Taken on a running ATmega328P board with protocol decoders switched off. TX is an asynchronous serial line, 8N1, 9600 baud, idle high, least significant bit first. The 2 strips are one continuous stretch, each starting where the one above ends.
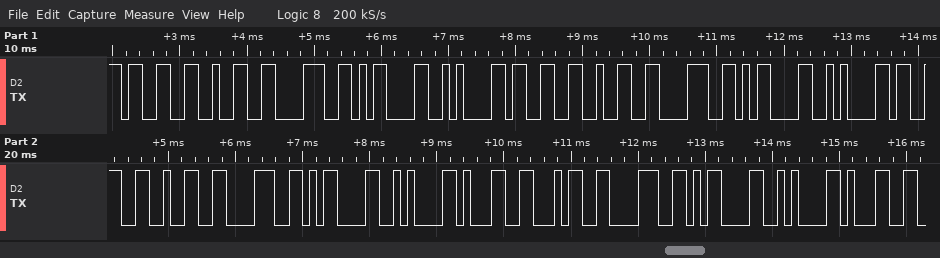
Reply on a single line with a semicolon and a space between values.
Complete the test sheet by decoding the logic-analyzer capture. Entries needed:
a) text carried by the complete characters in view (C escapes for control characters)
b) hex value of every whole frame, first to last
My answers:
"328\r\n328\r\n328\r\n148\r\n1"; 33 32 38 0D 0A 33 32 38 0D 0A 33 32 38 0D 0A 31 34 38 0D 0A 31
